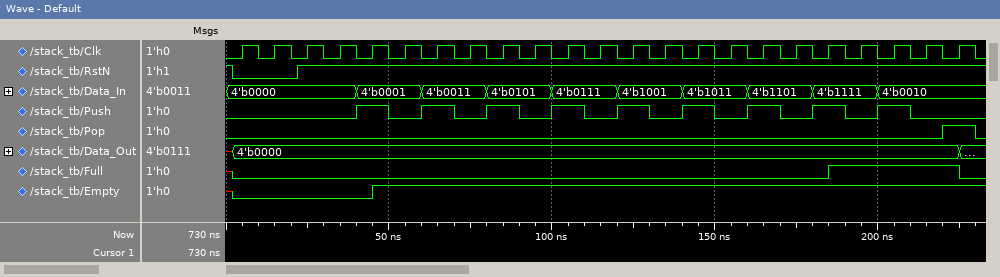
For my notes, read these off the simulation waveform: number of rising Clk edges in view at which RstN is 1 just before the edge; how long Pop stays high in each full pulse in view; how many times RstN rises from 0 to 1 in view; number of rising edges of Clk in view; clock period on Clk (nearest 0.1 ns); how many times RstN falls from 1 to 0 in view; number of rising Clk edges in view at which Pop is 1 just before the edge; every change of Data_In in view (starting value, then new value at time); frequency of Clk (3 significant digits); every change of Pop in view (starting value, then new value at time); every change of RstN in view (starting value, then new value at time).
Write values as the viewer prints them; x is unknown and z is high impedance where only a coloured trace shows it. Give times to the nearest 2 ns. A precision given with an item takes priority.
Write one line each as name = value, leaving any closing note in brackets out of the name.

number of rising Clk edges in view at which RstN is 1 just before the edge = 21
how long Pop stays high in each full pulse in view = 10 ns
how many times RstN rises from 0 to 1 in view = 1
number of rising edges of Clk in view = 23
clock period on Clk = 10 ns
how many times RstN falls from 1 to 0 in view = 1
number of rising Clk edges in view at which Pop is 1 just before the edge = 1
every change of Data_In in view = 4'b0000, 4'b0001 at 40 ns, 4'b0011 at 60 ns, 4'b0101 at 80 ns, 4'b0111 at 100 ns, 4'b1001 at 120 ns, 4'b1011 at 140 ns, 4'b1101 at 160 ns, 4'b1111 at 180 ns, 4'b0010 at 200 ns
frequency of Clk = 100 MHz
every change of Pop in view = 0, 1 at 220 ns, 0 at 230 ns
every change of RstN in view = 1, 0 at 2 ns, 1 at 22 ns
